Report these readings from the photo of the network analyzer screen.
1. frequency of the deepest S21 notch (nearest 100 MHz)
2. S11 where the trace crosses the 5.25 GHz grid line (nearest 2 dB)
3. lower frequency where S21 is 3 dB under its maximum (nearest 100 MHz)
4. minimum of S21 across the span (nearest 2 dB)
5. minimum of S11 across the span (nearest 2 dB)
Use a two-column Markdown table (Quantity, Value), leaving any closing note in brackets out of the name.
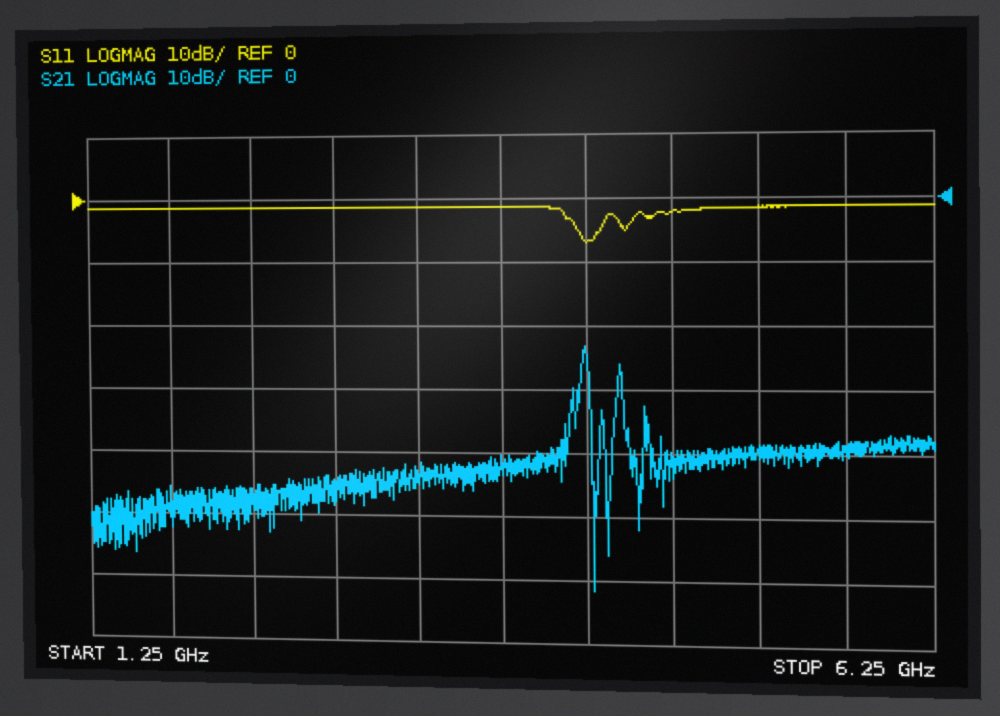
| Quantity | Value |
|---|---|
| frequency of the deepest S21 notch | 4.3 GHz |
| S11 where the trace crosses the 5.25 GHz grid line | -2 dB |
| lower frequency where S21 is 3 dB under its maximum | 4.2 GHz |
| minimum of S21 across the span | -62 dB |
| minimum of S11 across the span | -6 dB |
